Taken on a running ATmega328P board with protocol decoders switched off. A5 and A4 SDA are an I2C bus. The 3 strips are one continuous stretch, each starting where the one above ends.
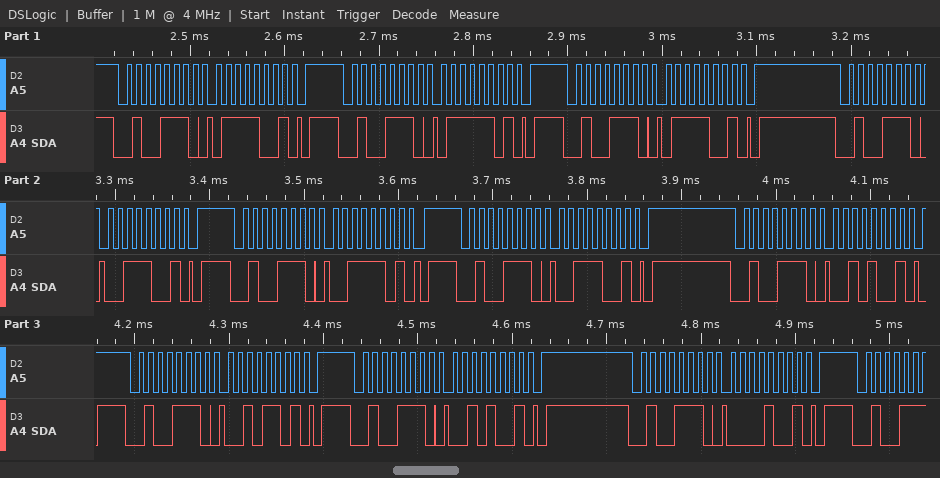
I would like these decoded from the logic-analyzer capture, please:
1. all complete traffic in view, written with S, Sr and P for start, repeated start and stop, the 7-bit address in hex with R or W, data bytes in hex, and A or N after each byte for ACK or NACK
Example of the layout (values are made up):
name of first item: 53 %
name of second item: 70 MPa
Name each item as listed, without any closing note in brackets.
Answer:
all complete traffic in view, written with S, Sr and P for start, repeated start and stop, the 7-bit address in hex with R or W, data bytes in hex, and A or N after each byte for ACK or NACK: S 27W A 79 A P S 27W A 7D A P S 27W A 79 A P S 27W A 39 A P S 27W A 3D A P S 27W A 39 A P S 27W A 29 A P S 27W A 2D A P S 27W A 29 A P S 27W A 09 A P
